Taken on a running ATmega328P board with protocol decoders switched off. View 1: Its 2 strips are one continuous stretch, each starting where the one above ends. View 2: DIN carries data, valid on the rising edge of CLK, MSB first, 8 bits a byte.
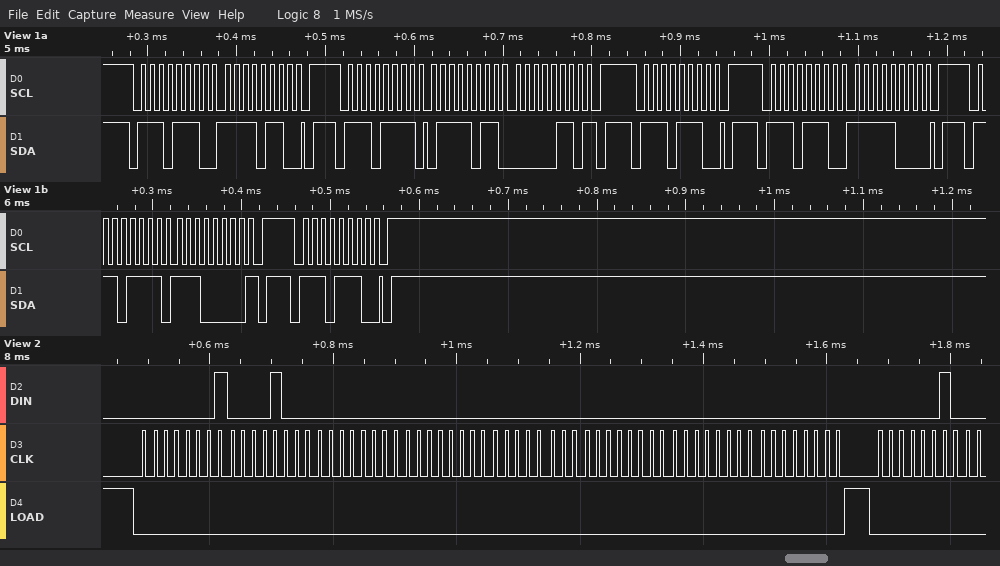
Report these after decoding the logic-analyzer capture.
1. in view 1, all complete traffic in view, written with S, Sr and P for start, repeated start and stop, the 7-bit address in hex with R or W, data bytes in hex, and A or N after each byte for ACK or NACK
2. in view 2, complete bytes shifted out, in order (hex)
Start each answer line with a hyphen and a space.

- S 77W A F6 A P S 77R A 7B A 06 N P S 77W A P S 77W A F8 A P S 77R A E0 N P S 77W A P
- 01 08 00 00 00 00 00 00 02
